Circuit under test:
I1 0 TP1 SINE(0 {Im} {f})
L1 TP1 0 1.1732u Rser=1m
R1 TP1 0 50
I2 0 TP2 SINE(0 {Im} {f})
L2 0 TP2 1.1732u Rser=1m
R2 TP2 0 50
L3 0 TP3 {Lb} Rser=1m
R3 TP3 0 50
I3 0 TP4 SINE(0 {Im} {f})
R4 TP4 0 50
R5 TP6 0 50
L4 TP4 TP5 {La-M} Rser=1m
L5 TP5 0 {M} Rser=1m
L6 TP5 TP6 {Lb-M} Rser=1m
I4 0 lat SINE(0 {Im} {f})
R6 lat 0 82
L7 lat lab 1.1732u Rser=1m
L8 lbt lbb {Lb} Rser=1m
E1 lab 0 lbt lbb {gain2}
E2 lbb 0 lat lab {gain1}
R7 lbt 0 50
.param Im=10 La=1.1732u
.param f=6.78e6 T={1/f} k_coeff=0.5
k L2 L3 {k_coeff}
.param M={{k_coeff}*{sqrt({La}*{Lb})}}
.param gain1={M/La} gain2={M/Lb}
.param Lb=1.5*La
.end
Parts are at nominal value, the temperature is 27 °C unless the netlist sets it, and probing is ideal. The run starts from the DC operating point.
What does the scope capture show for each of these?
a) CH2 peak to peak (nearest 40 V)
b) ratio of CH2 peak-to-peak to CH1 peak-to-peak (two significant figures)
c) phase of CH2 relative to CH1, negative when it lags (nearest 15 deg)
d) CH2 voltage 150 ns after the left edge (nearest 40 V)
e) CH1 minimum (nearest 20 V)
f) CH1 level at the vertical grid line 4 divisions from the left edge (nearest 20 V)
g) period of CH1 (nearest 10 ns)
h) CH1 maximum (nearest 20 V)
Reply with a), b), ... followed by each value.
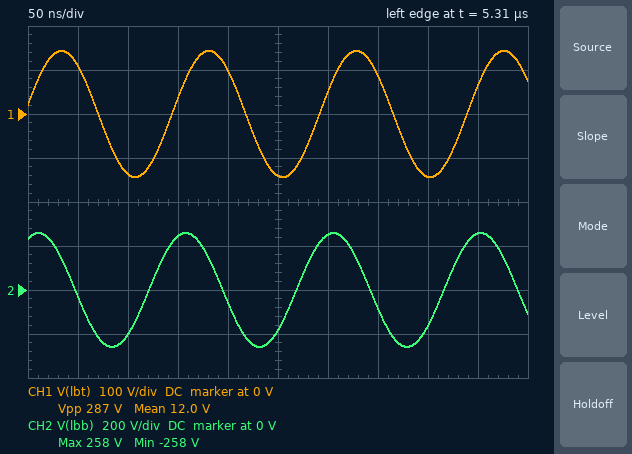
a) 520 V
b) 1.8
c) 60 deg
d) 240 V
e) -140 V
f) 100 V
g) 150 ns
h) 140 V
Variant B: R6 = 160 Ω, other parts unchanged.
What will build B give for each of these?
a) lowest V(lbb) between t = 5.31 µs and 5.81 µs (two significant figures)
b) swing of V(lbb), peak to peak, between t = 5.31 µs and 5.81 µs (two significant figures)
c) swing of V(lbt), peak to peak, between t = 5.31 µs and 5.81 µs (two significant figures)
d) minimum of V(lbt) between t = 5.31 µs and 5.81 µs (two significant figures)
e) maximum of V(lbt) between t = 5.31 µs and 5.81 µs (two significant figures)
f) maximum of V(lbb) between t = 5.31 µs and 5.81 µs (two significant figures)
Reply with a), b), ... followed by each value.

a) -290 V
b) 570 V
c) 320 V
d) -160 V
e) 160 V
f) 290 V
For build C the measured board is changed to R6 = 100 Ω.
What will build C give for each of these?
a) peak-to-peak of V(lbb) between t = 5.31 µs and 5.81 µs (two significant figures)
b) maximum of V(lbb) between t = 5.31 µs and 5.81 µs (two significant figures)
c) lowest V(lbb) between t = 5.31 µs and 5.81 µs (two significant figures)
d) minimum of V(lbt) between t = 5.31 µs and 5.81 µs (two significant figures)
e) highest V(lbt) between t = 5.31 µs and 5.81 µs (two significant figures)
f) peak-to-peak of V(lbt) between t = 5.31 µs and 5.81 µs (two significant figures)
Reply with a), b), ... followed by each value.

a) 540 V
b) 270 V
c) -270 V
d) -150 V
e) 150 V
f) 300 V
